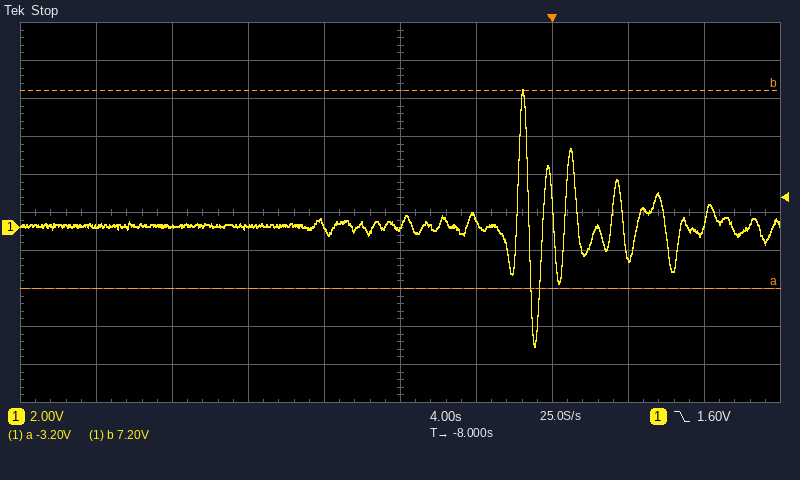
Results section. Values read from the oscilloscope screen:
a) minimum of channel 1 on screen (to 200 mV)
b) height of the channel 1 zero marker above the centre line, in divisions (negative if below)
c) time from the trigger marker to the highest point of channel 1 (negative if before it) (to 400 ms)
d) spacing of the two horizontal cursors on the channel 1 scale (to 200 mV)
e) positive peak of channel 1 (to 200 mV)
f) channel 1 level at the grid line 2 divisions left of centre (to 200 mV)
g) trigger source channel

-6.2 V
-0.4 div
-1.6 s
10.4 V
7.2 V
0.0 V
channel 1
